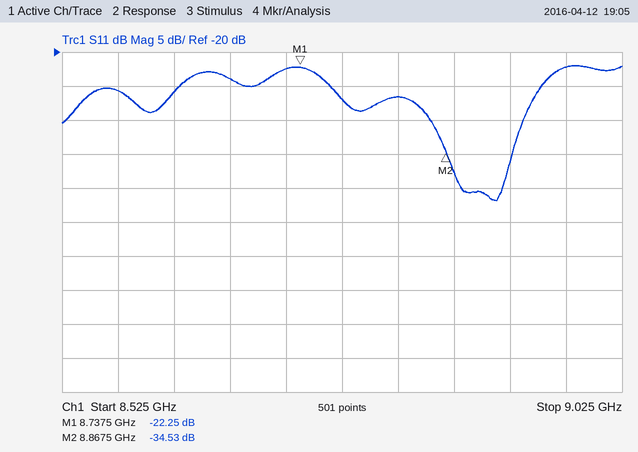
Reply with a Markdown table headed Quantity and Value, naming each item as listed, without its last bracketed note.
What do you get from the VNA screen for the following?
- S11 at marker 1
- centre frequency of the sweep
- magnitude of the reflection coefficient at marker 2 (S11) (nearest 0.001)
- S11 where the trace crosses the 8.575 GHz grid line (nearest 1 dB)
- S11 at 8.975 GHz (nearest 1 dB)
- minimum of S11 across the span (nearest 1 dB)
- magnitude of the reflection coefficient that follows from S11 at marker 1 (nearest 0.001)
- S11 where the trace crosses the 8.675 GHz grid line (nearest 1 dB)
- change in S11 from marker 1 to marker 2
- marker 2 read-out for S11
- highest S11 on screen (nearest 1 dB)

| Quantity | Value |
|---|---|
| S11 at marker 1 | -22.25 dB |
| centre frequency of the sweep | 8.775 GHz |
| magnitude of the reflection coefficient at marker 2 (S11) | 0.019 |
| S11 where the trace crosses the 8.575 GHz grid line | -26 dB |
| S11 at 8.975 GHz | -22 dB |
| minimum of S11 across the span | -42 dB |
| magnitude of the reflection coefficient that follows from S11 at marker 1 | 0.077 |
| S11 where the trace crosses the 8.675 GHz grid line | -24 dB |
| change in S11 from marker 1 to marker 2 | -12.28 dB |
| marker 2 read-out for S11 | -34.53 dB |
| highest S11 on screen | -22 dB |
